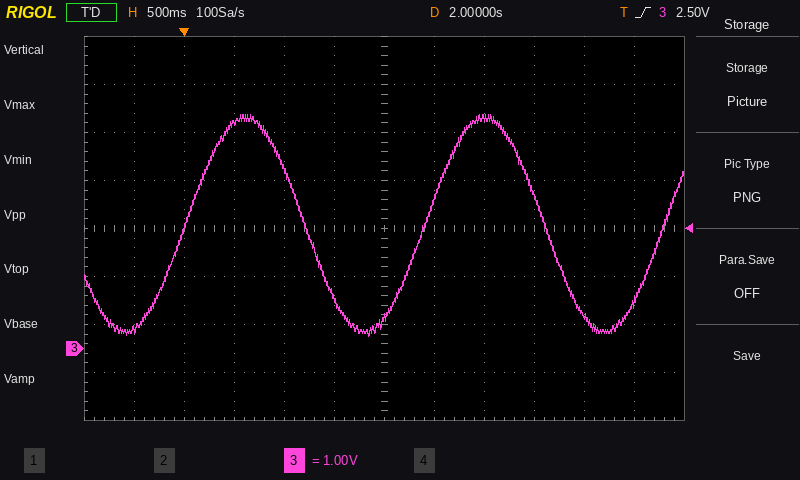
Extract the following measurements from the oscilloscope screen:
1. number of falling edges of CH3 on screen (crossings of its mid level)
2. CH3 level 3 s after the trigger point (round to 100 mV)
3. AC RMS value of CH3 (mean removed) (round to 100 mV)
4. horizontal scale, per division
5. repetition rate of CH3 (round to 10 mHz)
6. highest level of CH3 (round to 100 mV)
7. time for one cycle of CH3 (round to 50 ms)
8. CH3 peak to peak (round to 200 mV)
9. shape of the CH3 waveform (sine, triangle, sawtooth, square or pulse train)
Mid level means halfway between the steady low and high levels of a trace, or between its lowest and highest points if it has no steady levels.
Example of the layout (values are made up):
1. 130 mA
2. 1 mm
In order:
1. 2
2. 4.8 V
3. 1.6 V
4. 500 ms
5. 420 mHz
6. 4.9 V
7. 2.40 s
8. 4.6 V
9. sine
